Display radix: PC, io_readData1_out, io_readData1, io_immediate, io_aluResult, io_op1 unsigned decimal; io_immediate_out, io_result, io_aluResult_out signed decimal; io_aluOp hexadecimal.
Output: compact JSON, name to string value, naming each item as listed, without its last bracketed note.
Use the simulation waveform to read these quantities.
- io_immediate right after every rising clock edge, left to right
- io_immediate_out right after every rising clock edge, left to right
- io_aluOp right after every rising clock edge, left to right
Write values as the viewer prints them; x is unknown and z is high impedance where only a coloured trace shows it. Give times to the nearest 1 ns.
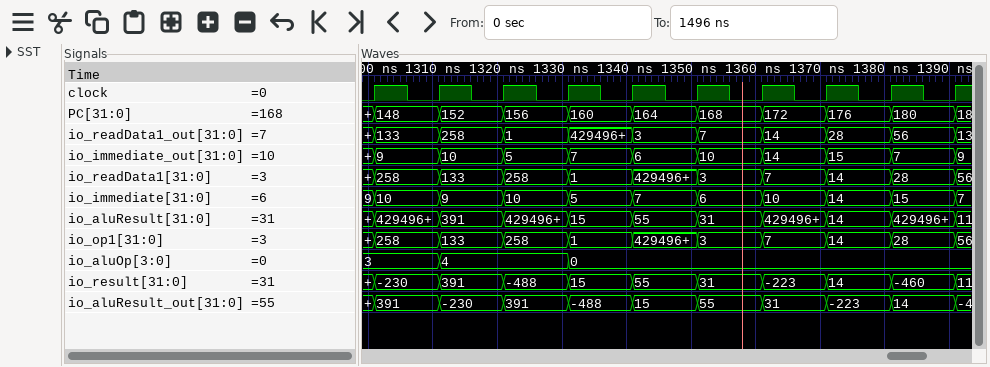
{"io_immediate right after every rising clock edge, left to right": "10, 9, 10, 5, 7, 6, 10, 14, 15, 7", "io_immediate_out right after every rising clock edge, left to right": "9, 10, 5, 7, 6, 10, 14, 15, 7, 9", "io_aluOp right after every rising clock edge, left to right": "3, 4, 4, 0, 0, 0, 0, 0, 0, 0"}
